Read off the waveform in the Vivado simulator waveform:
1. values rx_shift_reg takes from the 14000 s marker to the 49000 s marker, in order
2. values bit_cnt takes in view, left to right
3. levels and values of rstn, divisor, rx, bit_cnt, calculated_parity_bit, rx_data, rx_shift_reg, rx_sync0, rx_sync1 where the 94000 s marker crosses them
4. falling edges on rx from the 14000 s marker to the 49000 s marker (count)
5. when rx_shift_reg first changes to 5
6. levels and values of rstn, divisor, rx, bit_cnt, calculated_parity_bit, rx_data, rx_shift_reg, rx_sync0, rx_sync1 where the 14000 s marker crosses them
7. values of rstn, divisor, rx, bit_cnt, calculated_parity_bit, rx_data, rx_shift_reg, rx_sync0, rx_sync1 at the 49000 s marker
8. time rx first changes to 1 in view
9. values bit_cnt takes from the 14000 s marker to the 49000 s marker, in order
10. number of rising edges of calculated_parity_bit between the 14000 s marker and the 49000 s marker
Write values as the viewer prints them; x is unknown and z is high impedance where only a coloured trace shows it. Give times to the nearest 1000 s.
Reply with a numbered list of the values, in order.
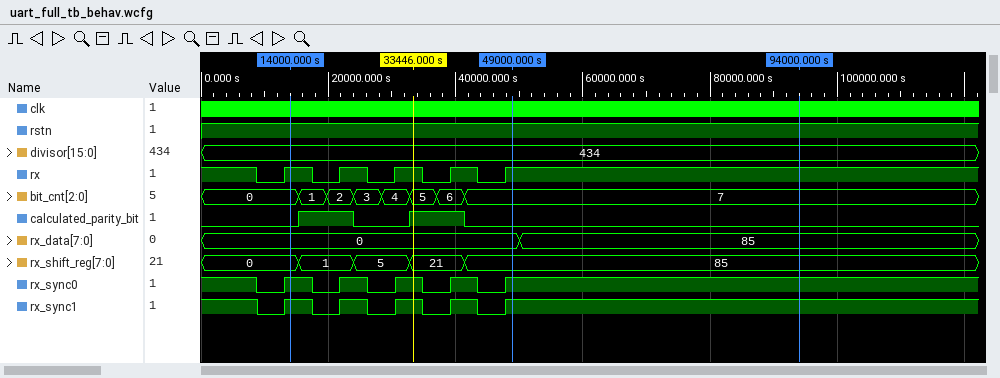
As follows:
1. 0, 1, 5, 21, 85
2. 0, 1, 2, 3, 4, 5, 6, 7
3. rstn=1, divisor=434, rx=1, bit_cnt=7, calculated_parity_bit=0, rx_data=85, rx_shift_reg=85, rx_sync0=1, rx_sync1=1
4. 4
5. 24000 s
6. rstn=1, divisor=434, rx=1, bit_cnt=0, calculated_parity_bit=0, rx_data=0, rx_shift_reg=0, rx_sync0=1, rx_sync1=1
7. rstn=1, divisor=434, rx=1, bit_cnt=7, calculated_parity_bit=0, rx_data=0, rx_shift_reg=85, rx_sync0=1, rx_sync1=1
8. 13000 s
9. 0, 1, 2, 3, 4, 5, 6, 7
10. 2
